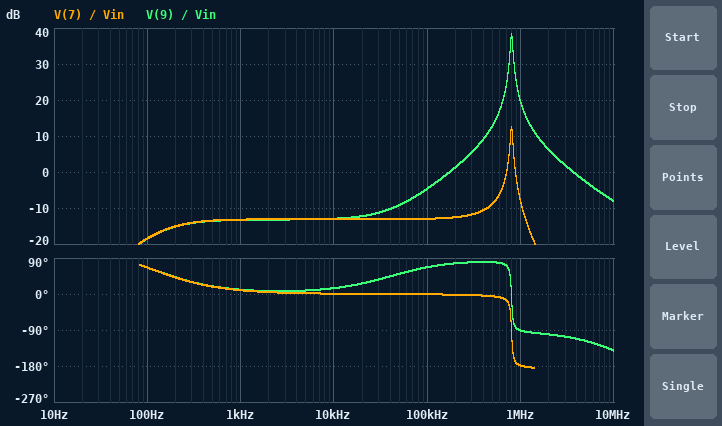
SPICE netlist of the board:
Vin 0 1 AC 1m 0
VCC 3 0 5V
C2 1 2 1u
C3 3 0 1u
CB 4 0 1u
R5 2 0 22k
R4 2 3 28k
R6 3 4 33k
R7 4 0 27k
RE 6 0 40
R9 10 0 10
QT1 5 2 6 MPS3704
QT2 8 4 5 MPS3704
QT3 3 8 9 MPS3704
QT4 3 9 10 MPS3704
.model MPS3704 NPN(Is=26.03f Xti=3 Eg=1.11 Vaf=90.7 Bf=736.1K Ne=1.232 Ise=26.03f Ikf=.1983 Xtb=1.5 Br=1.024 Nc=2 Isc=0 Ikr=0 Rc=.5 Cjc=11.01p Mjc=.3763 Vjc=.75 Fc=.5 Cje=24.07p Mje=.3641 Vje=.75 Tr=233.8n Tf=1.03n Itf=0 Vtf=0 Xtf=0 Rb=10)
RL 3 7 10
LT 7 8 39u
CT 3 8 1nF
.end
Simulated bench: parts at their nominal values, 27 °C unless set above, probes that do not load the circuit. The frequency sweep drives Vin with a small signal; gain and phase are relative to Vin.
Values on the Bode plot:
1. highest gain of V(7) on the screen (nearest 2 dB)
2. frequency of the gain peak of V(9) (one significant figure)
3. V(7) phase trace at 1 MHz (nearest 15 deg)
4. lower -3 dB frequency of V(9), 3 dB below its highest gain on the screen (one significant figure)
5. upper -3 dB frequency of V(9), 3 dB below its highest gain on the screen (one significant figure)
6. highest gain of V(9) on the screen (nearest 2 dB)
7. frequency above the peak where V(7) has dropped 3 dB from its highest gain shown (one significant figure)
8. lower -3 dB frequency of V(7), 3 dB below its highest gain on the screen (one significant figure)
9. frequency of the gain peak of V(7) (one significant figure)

12 dB
800 kHz
-180 deg
800 kHz
800 kHz
38 dB
800 kHz
800 kHz
800 kHz
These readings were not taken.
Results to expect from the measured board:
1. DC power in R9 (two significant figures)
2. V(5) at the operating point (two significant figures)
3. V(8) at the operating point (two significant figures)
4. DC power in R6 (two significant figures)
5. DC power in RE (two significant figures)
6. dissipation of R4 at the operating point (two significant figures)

1.2 W
570 mV
4.9 V
420 µW
4.1 mW
540 µW
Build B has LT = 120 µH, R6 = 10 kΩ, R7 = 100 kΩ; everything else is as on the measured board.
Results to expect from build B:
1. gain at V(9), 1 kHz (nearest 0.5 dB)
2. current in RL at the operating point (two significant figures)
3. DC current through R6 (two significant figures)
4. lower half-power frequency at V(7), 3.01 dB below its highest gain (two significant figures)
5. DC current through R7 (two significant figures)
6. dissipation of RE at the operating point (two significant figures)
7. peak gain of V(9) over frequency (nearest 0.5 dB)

-12.5 dB
12 mA
120 µA
450 kHz
38 µA
6.3 mW
48.0 dB
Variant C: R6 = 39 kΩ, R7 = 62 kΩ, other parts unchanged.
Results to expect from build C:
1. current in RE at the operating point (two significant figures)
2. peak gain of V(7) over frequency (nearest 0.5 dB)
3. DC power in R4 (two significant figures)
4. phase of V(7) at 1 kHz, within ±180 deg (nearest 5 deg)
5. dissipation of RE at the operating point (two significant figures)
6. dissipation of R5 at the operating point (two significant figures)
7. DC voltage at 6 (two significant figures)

11 mA
13.0 dB
530 µW
5 deg
5.1 mW
60 µW
450 mV
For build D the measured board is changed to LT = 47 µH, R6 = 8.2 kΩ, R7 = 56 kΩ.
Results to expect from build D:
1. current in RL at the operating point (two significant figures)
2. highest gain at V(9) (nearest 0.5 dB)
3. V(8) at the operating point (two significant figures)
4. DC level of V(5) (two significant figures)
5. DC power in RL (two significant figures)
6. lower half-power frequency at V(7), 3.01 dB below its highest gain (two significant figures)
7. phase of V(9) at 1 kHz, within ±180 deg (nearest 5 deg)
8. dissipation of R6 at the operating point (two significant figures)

12 mA
40.5 dB
4.9 V
3.1 V
1.5 mW
710 kHz
5 deg
180 µW
